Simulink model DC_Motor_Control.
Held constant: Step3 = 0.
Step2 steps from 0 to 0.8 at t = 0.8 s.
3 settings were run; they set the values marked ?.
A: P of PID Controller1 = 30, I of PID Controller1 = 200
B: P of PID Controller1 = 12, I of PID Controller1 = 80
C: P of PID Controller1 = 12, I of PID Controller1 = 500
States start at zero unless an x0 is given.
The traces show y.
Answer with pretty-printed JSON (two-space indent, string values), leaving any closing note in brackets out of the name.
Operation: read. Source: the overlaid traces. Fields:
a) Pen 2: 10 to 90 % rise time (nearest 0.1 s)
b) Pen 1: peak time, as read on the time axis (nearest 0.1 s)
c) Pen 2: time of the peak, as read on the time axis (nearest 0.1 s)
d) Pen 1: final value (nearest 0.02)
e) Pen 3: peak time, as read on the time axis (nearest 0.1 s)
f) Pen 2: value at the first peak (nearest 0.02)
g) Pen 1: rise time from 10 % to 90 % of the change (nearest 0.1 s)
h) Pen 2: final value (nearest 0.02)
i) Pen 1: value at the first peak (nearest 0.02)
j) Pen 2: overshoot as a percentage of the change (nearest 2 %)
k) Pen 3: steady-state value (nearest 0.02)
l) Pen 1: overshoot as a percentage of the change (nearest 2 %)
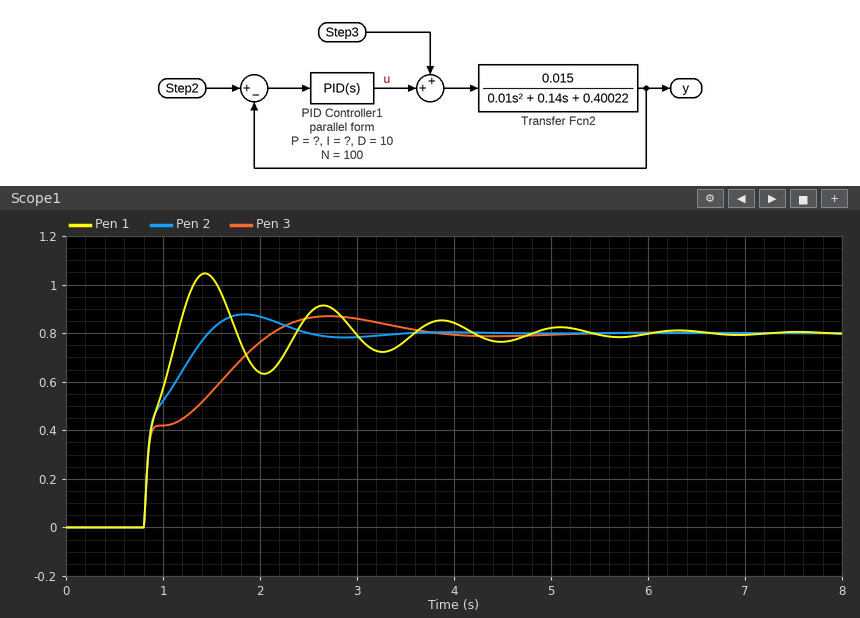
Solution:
{
  "Pen 2: 10 to 90 % rise time": "0.5 s",
  "Pen 1: peak time, as read on the time axis": "1.4 s",
  "Pen 2: time of the peak, as read on the time axis": "1.8 s",
  "Pen 1: final value": "0.80",
  "Pen 3: peak time, as read on the time axis": "2.7 s",
  "Pen 2: value at the first peak": "0.88",
  "Pen 1: rise time from 10 % to 90 % of the change": "0.3 s",
  "Pen 2: final value": "0.80",
  "Pen 1: value at the first peak": "1.04",
  "Pen 2: overshoot as a percentage of the change": "10 %",
  "Pen 3: steady-state value": "0.80",
  "Pen 1: overshoot as a percentage of the change": "30 %"
}
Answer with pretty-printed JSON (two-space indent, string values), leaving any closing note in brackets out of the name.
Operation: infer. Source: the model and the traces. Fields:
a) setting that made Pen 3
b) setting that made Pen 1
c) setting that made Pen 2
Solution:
{
  "setting that made Pen 3": "B",
  "setting that made Pen 1": "C",
  "setting that made Pen 2": "A"
}
